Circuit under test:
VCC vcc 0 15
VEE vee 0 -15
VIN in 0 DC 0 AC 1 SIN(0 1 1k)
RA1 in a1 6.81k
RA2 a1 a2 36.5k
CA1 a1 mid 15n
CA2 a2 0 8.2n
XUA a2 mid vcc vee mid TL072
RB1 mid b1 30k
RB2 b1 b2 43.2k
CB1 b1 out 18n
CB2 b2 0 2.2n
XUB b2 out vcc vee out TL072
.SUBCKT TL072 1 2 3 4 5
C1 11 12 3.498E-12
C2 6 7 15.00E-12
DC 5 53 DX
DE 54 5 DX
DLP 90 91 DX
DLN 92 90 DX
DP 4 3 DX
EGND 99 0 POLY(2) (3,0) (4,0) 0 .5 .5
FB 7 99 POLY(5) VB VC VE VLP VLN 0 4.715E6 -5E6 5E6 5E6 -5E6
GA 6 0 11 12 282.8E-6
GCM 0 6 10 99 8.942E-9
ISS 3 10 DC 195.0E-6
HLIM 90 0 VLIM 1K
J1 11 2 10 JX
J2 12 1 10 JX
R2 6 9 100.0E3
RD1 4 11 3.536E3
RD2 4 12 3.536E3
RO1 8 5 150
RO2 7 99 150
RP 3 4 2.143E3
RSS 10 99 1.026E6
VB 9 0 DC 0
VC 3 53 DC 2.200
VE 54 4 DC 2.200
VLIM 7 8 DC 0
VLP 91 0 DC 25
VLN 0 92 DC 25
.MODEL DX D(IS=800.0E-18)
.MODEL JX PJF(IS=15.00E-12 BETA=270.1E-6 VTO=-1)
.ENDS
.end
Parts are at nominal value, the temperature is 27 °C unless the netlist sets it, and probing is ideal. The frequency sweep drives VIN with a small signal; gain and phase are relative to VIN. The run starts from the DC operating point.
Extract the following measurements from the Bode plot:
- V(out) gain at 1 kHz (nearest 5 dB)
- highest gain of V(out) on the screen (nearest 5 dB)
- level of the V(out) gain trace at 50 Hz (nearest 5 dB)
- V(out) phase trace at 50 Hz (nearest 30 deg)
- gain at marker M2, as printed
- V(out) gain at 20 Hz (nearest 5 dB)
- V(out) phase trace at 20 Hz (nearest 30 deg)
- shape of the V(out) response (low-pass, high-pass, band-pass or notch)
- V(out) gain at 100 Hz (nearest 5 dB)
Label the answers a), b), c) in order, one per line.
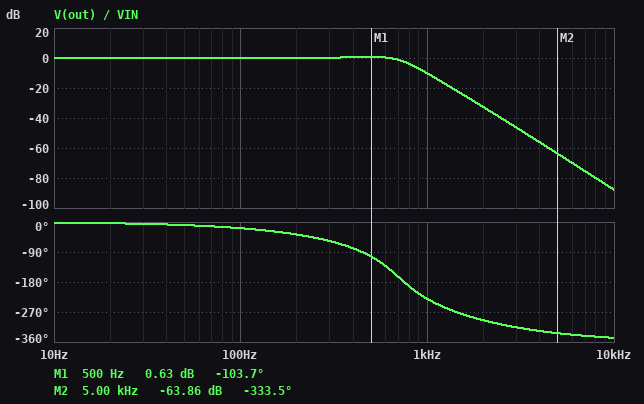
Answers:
a) -10 dB
b) 0 dB
c) 0 dB
d) 0 deg
e) -63.86 dB
f) 0 dB
g) 0 deg
h) low-pass
i) 0 dB
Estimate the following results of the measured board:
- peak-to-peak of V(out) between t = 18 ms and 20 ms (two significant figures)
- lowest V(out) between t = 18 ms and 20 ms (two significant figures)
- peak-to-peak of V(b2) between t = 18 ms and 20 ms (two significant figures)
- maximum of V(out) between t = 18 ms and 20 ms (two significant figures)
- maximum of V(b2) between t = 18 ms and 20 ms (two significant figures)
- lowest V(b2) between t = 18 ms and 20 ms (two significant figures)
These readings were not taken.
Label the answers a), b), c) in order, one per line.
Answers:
a) 620 mV
b) -310 mV
c) 620 mV
d) 310 mV
e) 310 mV
f) -310 mV
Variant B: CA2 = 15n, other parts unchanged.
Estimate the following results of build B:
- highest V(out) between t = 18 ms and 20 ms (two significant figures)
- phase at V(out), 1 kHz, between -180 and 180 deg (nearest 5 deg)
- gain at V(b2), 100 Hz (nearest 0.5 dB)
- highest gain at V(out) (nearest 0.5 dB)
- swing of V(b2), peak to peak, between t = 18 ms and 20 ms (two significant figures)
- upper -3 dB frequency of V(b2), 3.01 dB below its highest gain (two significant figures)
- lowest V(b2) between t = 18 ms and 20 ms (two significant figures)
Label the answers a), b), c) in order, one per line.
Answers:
a) 160 mV
b) 120 deg
c) -0.5 dB
d) 0 dB
e) 330 mV
f) 430 Hz
g) -160 mV
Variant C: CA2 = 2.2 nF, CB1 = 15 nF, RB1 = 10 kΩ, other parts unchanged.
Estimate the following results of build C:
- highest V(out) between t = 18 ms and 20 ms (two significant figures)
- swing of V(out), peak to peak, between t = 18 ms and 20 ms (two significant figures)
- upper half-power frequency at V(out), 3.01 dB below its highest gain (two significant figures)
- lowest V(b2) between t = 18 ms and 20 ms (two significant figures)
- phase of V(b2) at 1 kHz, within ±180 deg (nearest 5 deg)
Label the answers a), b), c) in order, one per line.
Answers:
a) 1.3 V
b) 2.6 V
c) 1.5 kHz
d) -1.3 V
e) -100 deg
